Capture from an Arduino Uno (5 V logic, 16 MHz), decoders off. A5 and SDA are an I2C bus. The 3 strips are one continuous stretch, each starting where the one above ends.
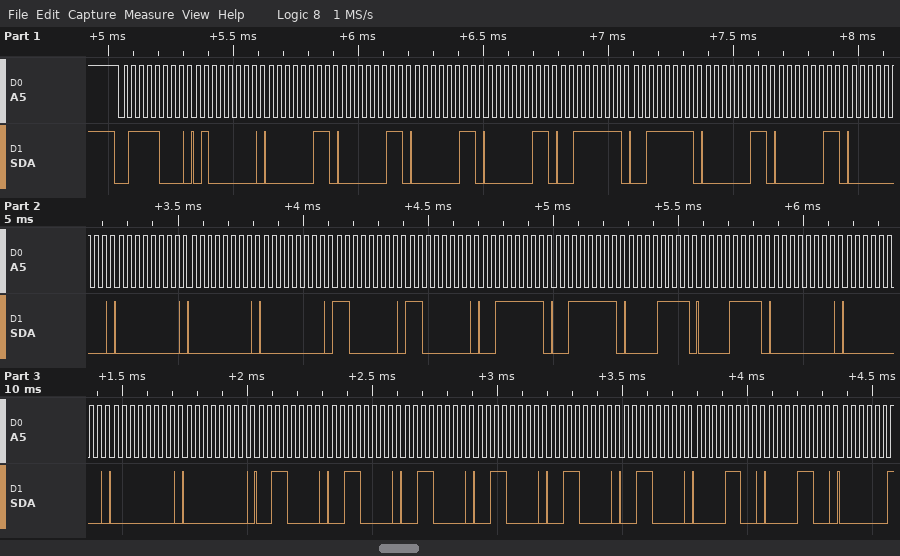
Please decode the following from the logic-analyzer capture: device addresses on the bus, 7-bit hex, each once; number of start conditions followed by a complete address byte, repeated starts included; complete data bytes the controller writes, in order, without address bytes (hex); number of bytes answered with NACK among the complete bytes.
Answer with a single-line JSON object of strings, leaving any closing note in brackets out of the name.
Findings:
{"device addresses on the bus, 7-bit hex, each once": "0x3C", "number of start conditions followed by a complete address byte, repeated starts included": "1", "complete data bytes the controller writes, in order, without address bytes": "40 03 03 03 03 3F 3F 03 03 00 00 00 00 C0 C0 3F 3F 0F 0F 00 00 00 00 30 30 30 30 30 30 0C 0C", "number of bytes answered with NACK among the complete bytes": "0"}
